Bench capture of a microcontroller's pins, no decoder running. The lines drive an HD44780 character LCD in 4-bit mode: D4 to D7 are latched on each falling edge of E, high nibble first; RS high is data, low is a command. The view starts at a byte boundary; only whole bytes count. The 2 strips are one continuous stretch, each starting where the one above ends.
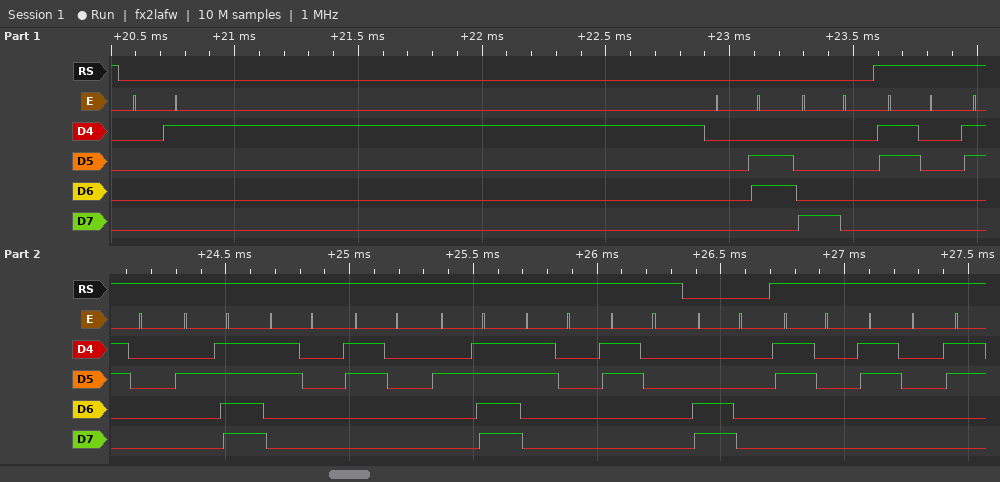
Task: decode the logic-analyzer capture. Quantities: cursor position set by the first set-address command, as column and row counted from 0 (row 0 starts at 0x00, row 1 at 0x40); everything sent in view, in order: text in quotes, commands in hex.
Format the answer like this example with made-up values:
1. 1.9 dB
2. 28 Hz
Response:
1. column 0, row 0
2. 0x01 0x06 0x80 "00/00/00" 0xC0 "00"
